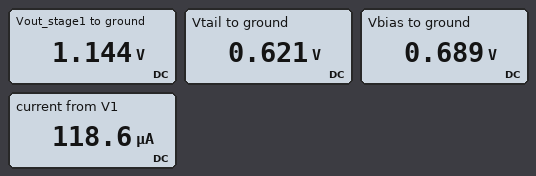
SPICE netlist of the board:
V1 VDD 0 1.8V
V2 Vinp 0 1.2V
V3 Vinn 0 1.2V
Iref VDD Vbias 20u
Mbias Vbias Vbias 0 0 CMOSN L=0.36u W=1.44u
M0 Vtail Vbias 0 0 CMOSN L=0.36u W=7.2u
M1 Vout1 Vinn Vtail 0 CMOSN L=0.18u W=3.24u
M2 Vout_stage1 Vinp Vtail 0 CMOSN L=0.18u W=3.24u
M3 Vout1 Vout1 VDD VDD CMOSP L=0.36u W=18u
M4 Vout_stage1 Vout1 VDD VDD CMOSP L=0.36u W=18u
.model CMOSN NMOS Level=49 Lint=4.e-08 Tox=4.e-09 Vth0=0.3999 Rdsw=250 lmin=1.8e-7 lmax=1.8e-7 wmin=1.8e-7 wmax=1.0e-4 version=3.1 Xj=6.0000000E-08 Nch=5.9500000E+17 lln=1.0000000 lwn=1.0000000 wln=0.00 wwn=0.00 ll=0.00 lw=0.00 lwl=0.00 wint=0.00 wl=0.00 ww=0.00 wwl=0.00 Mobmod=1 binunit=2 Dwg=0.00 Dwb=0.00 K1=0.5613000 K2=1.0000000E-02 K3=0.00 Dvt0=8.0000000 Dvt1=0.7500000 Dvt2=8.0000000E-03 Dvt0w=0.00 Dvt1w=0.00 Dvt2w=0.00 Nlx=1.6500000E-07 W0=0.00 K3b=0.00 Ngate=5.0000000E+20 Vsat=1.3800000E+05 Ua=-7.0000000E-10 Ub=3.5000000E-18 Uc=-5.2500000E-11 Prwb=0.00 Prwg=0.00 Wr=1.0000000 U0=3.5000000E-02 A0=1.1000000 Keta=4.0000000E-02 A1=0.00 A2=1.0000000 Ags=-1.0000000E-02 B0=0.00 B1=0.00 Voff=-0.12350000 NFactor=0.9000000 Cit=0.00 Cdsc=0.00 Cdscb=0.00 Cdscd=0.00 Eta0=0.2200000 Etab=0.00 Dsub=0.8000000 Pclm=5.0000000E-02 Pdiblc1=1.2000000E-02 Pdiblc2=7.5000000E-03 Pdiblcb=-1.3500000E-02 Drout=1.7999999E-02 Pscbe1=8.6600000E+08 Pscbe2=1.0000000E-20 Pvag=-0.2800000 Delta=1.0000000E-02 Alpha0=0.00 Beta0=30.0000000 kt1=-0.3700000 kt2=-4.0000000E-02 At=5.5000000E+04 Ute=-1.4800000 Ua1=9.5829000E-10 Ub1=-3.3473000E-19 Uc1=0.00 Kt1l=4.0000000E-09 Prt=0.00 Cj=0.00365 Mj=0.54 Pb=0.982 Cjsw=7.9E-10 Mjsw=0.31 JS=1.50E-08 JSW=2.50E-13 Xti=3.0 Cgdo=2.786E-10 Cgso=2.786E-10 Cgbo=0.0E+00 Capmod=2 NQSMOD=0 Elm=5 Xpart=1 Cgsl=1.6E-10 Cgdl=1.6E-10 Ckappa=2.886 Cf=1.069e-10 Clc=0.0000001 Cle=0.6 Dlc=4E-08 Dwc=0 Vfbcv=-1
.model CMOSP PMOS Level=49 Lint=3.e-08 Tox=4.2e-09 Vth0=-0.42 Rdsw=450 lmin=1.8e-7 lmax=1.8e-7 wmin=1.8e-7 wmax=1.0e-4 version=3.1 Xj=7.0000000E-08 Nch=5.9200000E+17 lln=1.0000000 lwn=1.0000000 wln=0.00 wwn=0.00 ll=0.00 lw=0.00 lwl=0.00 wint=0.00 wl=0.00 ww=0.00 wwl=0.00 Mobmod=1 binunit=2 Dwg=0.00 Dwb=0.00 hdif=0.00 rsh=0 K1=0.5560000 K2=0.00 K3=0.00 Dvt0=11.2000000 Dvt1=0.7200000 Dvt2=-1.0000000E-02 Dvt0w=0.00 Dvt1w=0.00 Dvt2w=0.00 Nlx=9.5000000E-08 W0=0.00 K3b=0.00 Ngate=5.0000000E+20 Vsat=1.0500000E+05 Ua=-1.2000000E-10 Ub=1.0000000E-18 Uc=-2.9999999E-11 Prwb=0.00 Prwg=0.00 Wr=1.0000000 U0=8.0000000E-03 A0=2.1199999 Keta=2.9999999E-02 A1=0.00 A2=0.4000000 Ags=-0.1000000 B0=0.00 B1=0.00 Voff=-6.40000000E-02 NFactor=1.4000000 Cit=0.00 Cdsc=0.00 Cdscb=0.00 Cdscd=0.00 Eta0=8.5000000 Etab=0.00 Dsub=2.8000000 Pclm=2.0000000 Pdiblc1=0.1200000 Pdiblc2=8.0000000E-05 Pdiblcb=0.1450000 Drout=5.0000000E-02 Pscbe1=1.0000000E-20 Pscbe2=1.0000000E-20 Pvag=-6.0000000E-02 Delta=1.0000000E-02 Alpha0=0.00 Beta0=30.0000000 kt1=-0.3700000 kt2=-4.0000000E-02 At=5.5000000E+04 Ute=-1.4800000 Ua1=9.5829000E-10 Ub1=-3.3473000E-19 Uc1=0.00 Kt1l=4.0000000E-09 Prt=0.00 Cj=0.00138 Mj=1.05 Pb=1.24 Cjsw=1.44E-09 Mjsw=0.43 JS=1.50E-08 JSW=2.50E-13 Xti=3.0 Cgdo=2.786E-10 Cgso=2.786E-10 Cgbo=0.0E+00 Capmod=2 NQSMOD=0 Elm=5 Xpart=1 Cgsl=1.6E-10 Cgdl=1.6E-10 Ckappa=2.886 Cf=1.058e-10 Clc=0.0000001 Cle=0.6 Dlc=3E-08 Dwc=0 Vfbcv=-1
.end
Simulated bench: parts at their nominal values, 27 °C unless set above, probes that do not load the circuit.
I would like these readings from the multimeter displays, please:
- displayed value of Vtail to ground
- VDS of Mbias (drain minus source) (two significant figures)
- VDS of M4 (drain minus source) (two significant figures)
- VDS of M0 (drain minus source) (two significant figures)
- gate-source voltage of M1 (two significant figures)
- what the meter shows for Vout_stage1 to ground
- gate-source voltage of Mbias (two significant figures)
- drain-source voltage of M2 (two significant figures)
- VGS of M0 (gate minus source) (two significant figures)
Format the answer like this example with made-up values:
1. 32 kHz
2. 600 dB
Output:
1. 0.621 V
2. 690 mV
3. -660 mV
4. 620 mV
5. 580 mV
6. 1.144 V
7. 690 mV
8. 520 mV
9. 690 mV
